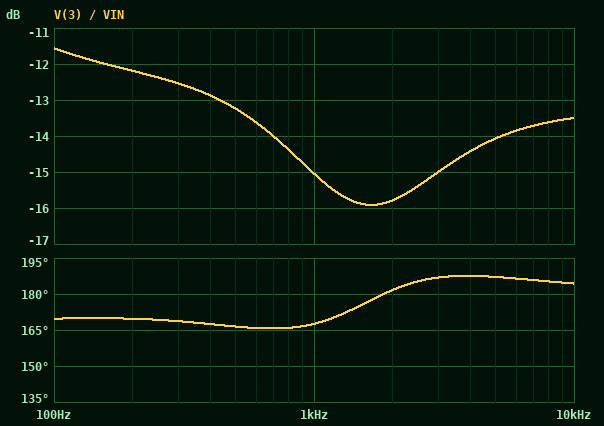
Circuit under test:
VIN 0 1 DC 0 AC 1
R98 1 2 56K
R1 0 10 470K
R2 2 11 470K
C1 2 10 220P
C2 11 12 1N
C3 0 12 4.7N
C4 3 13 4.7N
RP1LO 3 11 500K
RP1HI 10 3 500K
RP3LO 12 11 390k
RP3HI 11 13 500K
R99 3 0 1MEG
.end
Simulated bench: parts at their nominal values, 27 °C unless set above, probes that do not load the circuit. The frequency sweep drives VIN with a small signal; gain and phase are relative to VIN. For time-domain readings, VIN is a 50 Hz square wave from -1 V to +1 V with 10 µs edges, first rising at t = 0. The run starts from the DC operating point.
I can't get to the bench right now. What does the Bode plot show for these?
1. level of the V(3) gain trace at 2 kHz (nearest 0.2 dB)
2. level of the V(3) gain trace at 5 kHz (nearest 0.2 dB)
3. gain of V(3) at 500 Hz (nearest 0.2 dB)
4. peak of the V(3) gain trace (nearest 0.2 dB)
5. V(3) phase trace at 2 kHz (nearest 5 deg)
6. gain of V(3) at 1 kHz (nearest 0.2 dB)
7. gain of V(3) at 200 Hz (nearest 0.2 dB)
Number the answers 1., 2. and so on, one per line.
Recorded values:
1. -15.8 dB
2. -14.0 dB
3. -13.2 dB
4. -11.6 dB
5. 180 deg
6. -15.0 dB
7. -12.2 dB
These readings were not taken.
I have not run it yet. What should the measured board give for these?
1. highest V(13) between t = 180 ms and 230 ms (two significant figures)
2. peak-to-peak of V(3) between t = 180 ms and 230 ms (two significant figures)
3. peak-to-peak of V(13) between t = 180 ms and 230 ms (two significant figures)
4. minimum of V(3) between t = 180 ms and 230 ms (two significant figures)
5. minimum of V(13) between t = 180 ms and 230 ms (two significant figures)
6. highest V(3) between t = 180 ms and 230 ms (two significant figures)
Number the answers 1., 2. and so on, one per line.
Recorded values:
1. 560 mV
2. 640 mV
3. 1.1 V
4. -320 mV
5. -560 mV
6. 320 mV
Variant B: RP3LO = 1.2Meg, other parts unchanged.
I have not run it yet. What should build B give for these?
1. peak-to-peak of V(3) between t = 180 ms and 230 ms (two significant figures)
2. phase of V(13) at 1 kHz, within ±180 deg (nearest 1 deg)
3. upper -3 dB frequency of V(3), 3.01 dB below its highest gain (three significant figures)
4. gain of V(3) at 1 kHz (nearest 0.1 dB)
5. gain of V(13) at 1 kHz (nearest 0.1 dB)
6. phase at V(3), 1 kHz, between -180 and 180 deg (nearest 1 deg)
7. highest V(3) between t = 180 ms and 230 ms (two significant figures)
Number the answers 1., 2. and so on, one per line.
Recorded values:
1. 660 mV
2. 156 deg
3. 691 Hz
4. -14.6 dB
5. -15.0 dB
6. 158 deg
7. 330 mV
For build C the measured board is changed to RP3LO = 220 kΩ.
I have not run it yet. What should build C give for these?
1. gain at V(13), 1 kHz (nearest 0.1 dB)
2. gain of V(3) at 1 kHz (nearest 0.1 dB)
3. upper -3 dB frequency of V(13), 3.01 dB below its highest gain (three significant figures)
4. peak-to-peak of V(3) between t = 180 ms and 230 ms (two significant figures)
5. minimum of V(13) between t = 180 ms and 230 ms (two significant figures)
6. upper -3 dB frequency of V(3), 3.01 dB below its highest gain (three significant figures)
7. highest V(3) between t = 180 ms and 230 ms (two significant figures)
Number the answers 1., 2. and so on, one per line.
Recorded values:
1. -16.1 dB
2. -15.7 dB
3. 39.6 Hz
4. 650 mV
5. -570 mV
6. 129 Hz
7. 330 mV
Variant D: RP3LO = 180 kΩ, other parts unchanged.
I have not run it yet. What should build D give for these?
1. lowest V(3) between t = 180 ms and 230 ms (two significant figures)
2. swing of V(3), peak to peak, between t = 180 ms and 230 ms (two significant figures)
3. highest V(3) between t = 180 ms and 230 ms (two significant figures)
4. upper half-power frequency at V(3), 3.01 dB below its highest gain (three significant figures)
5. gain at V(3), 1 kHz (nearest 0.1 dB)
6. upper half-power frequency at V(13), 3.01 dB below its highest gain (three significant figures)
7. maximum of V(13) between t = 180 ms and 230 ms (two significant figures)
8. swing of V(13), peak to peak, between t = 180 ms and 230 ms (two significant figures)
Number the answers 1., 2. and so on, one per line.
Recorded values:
1. -330 mV
2. 660 mV
3. 330 mV
4. 120 Hz
5. -16.0 dB
6. 40.4 Hz
7. 570 mV
8. 1.1 V
